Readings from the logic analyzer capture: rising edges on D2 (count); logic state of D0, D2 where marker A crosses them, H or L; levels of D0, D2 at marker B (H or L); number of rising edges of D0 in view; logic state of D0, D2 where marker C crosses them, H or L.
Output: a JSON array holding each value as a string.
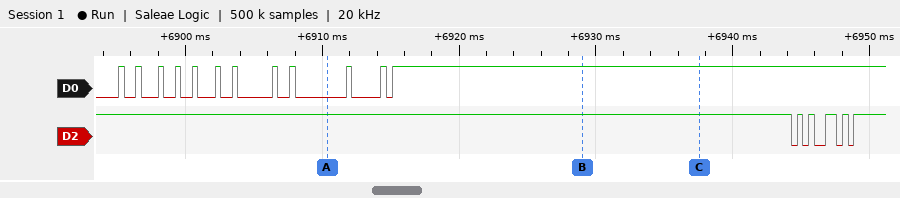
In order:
["5", "D0=L, D2=H", "D0=H, D2=H", "12", "D0=H, D2=H"]
